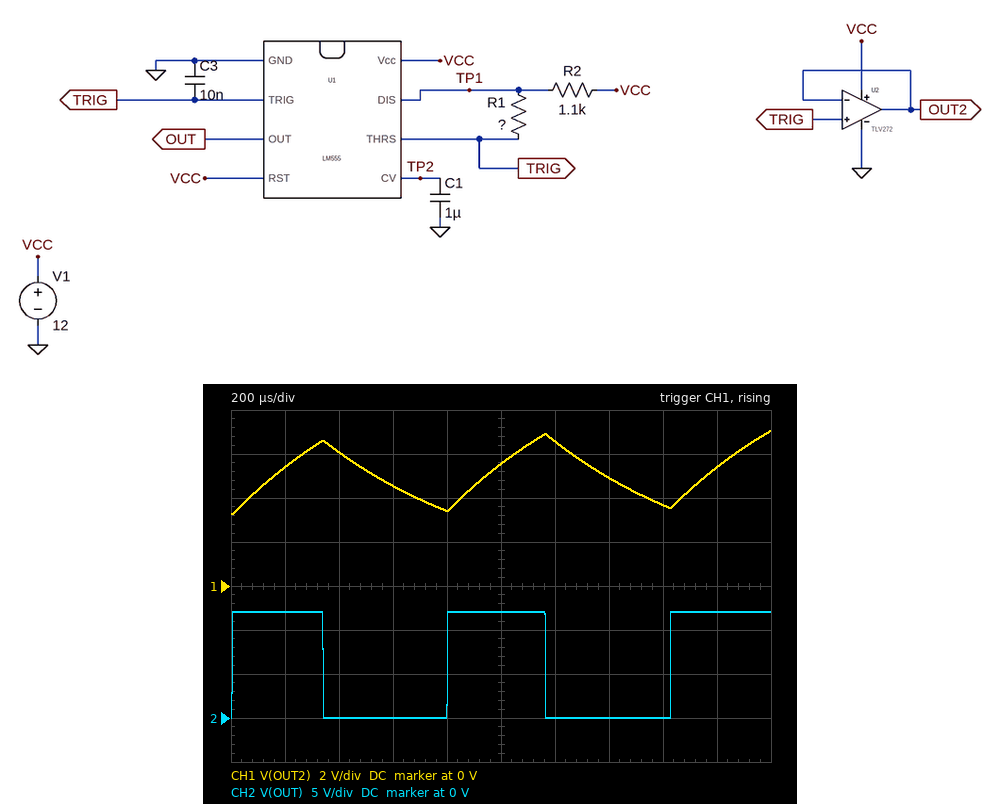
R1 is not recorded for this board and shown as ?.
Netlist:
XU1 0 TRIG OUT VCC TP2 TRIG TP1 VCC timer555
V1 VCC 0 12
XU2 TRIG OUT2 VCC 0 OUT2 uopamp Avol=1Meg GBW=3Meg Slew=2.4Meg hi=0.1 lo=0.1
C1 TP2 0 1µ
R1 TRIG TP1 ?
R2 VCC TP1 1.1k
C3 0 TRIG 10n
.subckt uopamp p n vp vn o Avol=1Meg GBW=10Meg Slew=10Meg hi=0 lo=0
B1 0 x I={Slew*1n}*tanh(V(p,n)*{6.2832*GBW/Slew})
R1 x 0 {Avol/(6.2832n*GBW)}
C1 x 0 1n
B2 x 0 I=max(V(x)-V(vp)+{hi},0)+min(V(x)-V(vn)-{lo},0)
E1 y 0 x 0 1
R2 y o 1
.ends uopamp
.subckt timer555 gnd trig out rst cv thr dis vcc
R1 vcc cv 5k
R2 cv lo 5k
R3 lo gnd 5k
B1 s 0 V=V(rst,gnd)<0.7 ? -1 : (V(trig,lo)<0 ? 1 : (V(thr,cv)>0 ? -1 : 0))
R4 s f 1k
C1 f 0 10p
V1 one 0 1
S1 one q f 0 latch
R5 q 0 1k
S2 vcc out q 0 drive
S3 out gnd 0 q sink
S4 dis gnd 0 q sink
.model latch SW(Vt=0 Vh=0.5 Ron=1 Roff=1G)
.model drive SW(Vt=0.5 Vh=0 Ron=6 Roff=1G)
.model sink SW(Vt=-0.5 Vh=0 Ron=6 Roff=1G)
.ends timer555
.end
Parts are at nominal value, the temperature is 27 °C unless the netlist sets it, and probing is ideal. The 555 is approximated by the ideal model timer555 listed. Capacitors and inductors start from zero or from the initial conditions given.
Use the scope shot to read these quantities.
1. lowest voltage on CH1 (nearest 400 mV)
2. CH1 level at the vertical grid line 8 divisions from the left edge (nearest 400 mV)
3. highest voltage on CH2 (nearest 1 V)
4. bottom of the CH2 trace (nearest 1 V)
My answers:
3.2 V
3.6 V
12 V
0 V
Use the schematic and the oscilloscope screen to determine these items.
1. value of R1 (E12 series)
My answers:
68 kΩ
